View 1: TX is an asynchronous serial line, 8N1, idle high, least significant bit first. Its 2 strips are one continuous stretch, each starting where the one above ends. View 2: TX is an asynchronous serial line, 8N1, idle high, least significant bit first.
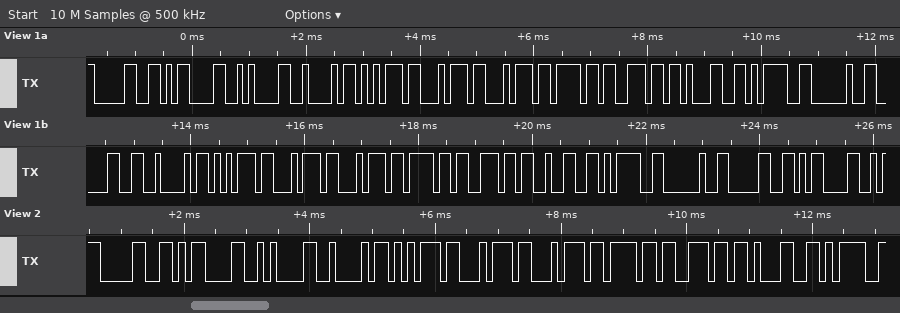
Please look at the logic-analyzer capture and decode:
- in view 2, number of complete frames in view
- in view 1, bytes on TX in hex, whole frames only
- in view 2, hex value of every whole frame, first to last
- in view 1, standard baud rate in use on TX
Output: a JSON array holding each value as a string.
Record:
["11", "0x30 0x0D 0x0A 0x42 0x75 0x74 0x74 0x6F 0x6E 0x31 0x3D 0x20 0x30 0x42 0x75 0x74 0x74 0x6F 0x6E 0x32 0x3D 0x20 0x30 0x0D", "0x30 0x0D 0x0A 0x42 0x75 0x74 0x74 0x6F 0x6E 0x31 0x3D", "9600 baud"]
